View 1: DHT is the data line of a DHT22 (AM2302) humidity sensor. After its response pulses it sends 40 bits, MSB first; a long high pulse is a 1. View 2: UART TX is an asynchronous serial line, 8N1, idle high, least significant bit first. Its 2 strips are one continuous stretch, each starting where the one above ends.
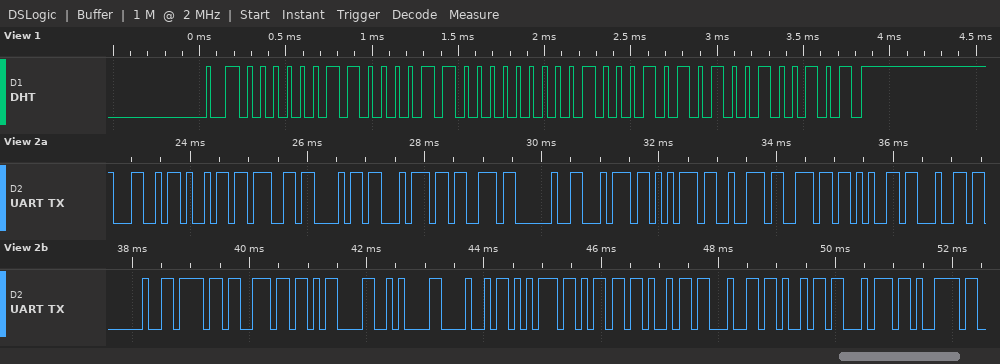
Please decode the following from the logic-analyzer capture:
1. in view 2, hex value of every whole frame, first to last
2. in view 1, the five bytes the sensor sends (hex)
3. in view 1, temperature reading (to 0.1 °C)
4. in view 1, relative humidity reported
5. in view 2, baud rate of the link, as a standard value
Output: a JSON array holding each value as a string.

["4C 69 67 68 74 73 20 74 75 72 6E 65 64 20 6F 6E 0D 0A 48 75 6D 69 64 69 74 79", "03 0C 01 15 25", "27.7 °C", "78.0 %", "9600 baud"]
